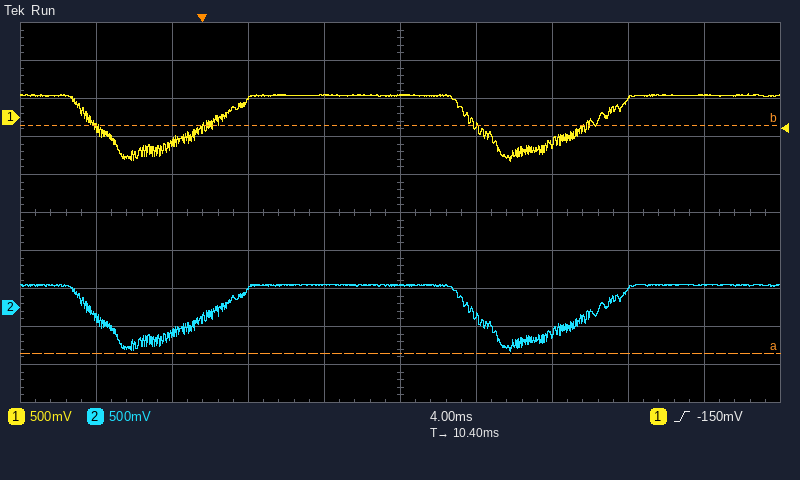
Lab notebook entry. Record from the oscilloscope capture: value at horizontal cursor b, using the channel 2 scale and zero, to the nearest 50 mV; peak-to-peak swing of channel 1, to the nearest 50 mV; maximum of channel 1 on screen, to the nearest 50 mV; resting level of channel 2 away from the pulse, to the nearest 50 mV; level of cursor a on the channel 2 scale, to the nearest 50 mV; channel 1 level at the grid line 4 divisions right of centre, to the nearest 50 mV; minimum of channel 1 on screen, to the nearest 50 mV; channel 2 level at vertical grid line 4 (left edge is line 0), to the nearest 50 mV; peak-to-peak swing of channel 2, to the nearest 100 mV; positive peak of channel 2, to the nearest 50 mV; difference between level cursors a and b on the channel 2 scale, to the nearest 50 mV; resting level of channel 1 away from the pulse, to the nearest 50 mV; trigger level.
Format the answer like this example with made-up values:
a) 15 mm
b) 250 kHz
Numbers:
a) 2.40 V
b) 900 mV
c) 300 mV
d) 300 mV
e) -600 mV
f) 300 mV
g) -600 mV
h) 300 mV
i) 900 mV
j) 300 mV
k) 3.00 V
l) 300 mV
m) -150 mV
